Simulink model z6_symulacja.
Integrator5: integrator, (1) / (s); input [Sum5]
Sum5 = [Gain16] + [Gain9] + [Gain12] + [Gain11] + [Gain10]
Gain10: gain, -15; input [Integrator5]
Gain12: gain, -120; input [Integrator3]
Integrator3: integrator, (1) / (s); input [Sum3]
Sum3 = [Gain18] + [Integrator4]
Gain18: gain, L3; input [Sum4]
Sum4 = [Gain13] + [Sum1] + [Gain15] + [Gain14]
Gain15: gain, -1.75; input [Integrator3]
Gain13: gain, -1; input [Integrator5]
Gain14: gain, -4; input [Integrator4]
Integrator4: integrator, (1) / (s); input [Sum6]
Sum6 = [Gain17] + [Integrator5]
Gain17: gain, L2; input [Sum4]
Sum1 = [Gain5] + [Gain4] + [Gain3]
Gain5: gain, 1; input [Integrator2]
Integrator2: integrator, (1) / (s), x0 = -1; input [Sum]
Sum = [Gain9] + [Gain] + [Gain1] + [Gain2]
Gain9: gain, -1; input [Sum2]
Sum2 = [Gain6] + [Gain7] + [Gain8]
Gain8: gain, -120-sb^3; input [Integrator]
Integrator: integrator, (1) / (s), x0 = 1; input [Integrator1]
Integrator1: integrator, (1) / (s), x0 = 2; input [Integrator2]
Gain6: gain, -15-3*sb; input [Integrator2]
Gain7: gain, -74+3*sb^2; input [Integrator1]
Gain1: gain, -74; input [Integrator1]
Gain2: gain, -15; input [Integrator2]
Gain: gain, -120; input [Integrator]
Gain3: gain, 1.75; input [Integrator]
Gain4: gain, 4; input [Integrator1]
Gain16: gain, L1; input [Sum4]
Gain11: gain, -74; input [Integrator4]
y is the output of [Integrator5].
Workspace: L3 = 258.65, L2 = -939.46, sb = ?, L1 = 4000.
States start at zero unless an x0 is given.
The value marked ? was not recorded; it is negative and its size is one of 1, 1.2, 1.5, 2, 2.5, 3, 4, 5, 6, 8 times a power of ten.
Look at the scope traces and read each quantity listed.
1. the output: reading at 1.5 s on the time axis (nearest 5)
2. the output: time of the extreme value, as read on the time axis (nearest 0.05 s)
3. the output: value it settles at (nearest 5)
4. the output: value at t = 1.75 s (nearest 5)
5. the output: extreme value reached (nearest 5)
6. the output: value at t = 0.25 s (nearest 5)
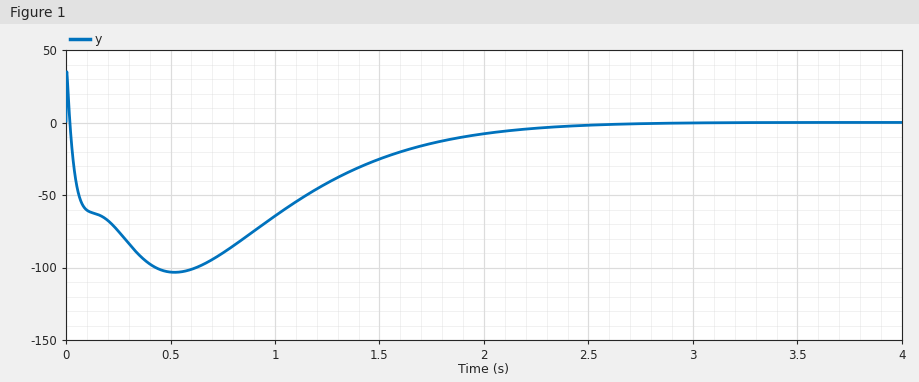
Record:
-25
0.50 s
0
-15
-105
-75
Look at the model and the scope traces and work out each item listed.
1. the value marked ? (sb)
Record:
-12
